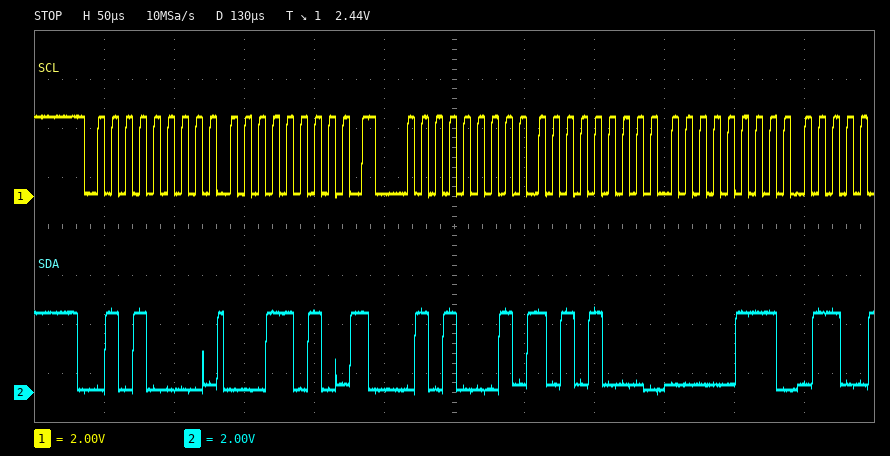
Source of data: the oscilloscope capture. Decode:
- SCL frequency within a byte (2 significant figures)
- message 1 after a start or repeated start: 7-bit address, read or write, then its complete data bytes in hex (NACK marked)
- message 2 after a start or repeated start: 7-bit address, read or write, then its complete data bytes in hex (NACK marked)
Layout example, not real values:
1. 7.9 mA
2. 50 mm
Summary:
1. 100 kHz
2. 0x28 write: 1A
3. 0x28 read: A8 07
